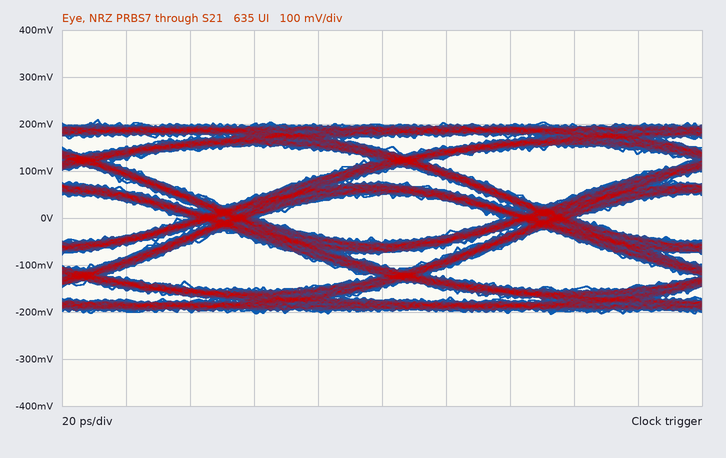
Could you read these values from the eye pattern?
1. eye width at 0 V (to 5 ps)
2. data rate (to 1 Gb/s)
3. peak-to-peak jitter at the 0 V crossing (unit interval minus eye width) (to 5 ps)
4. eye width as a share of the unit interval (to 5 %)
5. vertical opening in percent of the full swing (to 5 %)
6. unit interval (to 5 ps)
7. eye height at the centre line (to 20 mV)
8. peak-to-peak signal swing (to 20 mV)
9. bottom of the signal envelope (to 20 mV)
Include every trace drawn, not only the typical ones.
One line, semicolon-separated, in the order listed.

75 ps; 10 Gb/s; 25 ps; 75 %; 25 %; 100 ps; 100 mV; 420 mV; -200 mV
